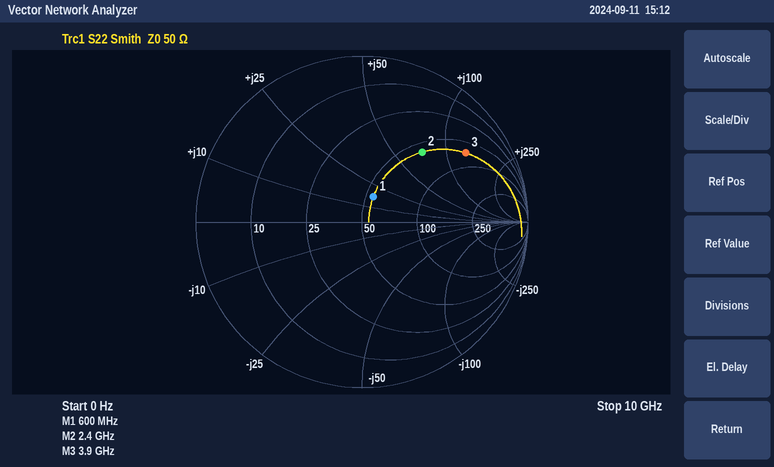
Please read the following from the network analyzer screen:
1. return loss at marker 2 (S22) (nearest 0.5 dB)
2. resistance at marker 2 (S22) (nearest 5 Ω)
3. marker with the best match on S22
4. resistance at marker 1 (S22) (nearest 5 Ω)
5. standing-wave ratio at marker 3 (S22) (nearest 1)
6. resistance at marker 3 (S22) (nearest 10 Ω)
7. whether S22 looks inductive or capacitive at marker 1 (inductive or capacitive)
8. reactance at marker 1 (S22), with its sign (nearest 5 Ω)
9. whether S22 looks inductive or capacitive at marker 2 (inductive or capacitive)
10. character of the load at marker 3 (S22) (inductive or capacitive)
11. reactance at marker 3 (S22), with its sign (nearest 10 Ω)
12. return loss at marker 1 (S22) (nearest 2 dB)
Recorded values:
5.0 dB
60 Ω
marker 1
55 Ω
7
70 Ω
inductive
+15 Ω
inductive
inductive
+130 Ω
16 dB
